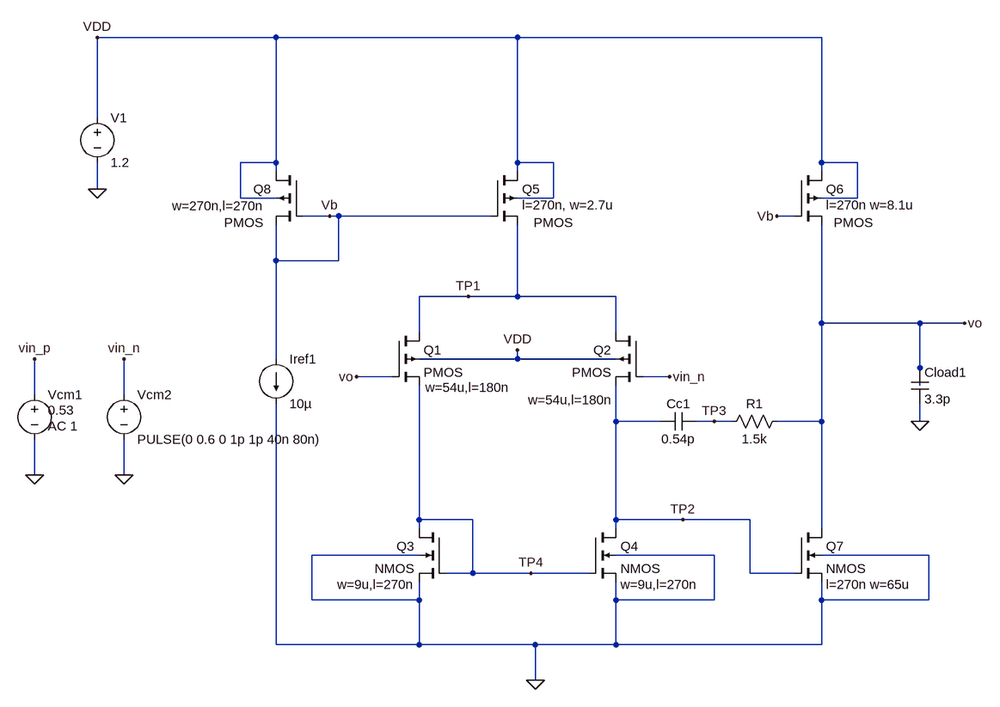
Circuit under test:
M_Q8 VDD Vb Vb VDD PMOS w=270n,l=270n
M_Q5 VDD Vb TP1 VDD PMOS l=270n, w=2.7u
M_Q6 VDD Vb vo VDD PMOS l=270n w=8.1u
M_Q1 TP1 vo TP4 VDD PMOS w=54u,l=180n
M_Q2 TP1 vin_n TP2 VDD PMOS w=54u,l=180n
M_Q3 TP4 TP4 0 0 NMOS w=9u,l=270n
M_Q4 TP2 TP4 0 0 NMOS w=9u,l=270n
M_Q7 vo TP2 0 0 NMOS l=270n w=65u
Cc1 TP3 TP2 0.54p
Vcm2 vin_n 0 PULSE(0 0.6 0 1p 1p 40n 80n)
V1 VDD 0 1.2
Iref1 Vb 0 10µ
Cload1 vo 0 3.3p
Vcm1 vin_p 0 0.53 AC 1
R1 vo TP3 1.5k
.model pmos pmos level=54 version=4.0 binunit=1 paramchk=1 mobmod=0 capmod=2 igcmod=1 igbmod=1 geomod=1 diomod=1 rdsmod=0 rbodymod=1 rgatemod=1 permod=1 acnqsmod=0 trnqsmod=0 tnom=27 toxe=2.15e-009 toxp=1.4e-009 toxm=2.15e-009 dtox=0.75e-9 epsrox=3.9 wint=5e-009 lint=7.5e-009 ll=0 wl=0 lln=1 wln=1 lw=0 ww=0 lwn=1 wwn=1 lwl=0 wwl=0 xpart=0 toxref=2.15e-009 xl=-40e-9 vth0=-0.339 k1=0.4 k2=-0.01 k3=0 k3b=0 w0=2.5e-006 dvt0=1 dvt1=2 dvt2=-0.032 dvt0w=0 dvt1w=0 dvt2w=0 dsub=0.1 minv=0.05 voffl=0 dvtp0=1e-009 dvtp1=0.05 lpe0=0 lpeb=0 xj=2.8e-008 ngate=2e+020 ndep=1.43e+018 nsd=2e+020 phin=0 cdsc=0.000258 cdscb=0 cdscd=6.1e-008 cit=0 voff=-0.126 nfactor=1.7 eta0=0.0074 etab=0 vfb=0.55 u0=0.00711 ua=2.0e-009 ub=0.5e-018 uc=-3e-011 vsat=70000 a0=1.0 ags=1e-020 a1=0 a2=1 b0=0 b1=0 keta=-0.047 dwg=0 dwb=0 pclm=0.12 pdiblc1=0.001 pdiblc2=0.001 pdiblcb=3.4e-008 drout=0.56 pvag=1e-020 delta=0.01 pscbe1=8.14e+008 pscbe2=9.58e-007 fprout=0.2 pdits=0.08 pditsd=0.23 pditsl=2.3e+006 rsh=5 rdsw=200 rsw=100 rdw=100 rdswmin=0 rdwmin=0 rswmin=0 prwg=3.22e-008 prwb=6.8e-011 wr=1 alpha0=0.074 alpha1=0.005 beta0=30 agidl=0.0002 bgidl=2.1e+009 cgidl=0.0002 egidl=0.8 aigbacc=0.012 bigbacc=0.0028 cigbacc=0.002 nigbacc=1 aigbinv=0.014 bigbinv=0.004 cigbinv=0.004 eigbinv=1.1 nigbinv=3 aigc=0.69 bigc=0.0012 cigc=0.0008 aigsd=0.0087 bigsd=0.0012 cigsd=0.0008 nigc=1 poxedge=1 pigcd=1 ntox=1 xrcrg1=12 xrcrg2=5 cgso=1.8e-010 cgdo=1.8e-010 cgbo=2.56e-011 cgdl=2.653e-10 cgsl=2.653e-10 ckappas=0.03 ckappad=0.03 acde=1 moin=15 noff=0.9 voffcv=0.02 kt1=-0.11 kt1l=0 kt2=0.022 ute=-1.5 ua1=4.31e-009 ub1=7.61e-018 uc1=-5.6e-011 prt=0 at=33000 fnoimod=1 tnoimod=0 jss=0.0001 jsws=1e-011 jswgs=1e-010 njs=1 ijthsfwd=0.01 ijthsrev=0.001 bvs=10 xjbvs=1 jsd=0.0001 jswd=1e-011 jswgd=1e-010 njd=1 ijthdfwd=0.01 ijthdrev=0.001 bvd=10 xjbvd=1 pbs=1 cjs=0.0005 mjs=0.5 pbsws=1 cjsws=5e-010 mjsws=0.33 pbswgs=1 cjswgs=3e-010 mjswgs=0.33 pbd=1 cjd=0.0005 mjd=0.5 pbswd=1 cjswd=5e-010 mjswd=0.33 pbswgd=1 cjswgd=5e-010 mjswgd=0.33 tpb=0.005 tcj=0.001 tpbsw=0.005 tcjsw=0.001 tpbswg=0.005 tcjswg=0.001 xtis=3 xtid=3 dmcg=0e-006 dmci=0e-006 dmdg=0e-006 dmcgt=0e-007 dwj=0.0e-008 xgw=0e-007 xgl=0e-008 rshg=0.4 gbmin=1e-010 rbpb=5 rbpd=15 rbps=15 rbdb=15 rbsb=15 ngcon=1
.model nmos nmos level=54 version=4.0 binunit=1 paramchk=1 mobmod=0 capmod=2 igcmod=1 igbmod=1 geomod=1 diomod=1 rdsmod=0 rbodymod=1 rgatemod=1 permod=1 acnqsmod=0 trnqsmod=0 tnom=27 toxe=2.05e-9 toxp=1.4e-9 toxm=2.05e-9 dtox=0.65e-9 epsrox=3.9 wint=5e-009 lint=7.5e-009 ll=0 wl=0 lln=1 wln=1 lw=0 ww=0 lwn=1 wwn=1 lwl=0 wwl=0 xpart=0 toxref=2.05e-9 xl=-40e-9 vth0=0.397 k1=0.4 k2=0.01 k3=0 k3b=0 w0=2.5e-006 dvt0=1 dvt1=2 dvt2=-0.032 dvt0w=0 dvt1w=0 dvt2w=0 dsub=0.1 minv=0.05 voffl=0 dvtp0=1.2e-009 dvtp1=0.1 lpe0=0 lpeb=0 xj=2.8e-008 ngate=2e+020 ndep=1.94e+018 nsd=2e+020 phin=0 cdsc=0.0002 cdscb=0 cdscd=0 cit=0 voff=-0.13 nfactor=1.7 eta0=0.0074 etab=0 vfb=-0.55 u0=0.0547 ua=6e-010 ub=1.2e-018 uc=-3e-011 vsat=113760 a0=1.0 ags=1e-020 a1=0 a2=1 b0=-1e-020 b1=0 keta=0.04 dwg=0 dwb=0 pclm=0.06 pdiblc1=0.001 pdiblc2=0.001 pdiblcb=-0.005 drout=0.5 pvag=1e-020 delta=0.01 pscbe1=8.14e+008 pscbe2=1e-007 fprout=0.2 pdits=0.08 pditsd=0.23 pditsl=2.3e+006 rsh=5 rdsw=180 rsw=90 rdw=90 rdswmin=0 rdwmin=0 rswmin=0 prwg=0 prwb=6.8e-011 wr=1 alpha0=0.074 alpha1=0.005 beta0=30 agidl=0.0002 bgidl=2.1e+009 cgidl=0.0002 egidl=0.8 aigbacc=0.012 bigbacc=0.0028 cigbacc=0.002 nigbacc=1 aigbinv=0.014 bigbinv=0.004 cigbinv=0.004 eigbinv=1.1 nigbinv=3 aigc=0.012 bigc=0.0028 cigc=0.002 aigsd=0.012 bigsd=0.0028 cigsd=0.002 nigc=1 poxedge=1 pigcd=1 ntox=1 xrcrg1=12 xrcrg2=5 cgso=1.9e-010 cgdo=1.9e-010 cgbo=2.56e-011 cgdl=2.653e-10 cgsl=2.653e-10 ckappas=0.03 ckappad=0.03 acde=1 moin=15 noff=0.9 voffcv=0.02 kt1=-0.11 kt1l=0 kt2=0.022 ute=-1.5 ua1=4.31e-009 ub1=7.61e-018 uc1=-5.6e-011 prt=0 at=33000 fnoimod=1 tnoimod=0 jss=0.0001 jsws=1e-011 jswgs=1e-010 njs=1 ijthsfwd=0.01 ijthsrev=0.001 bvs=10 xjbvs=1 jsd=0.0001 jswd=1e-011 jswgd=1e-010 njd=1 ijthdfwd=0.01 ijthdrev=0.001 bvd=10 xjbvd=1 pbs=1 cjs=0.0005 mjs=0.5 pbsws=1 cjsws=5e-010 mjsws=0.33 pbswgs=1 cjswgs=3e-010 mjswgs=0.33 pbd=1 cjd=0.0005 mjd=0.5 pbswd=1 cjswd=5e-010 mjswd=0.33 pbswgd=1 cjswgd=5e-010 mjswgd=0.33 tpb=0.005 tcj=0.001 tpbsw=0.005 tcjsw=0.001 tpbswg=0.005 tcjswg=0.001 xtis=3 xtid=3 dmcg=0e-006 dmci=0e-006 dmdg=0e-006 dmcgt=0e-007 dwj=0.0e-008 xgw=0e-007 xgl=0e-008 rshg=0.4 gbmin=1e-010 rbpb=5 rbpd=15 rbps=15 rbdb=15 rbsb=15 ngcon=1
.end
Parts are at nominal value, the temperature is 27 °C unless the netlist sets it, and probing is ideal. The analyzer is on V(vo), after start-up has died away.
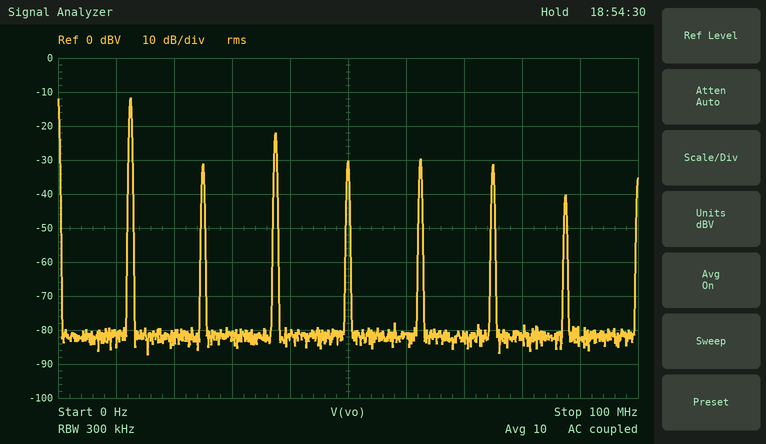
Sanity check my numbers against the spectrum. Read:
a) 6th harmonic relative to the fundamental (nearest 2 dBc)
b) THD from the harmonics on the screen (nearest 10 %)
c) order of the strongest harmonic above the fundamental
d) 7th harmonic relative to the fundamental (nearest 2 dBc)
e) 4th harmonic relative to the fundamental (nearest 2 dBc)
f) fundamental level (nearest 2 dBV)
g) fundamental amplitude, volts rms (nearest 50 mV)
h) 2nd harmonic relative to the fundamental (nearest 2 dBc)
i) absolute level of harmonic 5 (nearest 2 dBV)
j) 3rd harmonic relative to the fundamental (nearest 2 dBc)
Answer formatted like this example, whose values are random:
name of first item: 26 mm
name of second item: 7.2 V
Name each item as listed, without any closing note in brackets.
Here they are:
6th harmonic relative to the fundamental: -20 dBc
THD from the harmonics on the screen: 40 %
order of the strongest harmonic above the fundamental: 3
7th harmonic relative to the fundamental: -28 dBc
4th harmonic relative to the fundamental: -18 dBc
fundamental level: -12 dBV
fundamental amplitude, volts rms: 250 mV
2nd harmonic relative to the fundamental: -20 dBc
absolute level of harmonic 5: -30 dBV
3rd harmonic relative to the fundamental: -10 dBc
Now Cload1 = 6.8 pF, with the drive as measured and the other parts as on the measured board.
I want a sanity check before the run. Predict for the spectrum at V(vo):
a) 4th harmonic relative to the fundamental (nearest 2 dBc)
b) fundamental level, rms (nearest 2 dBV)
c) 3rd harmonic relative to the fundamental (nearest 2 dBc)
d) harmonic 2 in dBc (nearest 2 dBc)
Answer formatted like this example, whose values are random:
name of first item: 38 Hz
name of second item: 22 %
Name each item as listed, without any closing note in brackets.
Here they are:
4th harmonic relative to the fundamental: -16 dBc
fundamental level, rms: -12 dBV
3rd harmonic relative to the fundamental: -14 dBc
harmonic 2 in dBc: -12 dBc
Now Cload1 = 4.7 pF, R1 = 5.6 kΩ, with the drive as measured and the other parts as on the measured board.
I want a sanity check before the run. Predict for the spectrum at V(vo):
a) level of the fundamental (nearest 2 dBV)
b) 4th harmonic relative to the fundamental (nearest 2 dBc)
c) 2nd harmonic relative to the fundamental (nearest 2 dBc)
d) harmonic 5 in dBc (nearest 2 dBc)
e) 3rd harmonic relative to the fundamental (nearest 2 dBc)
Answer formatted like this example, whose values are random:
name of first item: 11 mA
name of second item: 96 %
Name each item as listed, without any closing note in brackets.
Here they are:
level of the fundamental: -12 dBV
4th harmonic relative to the fundamental: -16 dBc
2nd harmonic relative to the fundamental: -16 dBc
harmonic 5 in dBc: -22 dBc
3rd harmonic relative to the fundamental: -12 dBc
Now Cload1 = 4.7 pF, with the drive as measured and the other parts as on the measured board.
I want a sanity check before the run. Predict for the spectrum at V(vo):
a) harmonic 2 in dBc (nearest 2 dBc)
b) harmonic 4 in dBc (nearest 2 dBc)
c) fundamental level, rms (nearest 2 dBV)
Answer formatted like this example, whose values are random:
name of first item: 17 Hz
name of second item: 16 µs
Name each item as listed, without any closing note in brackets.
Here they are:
harmonic 2 in dBc: -16 dBc
harmonic 4 in dBc: -16 dBc
fundamental level, rms: -12 dBV
